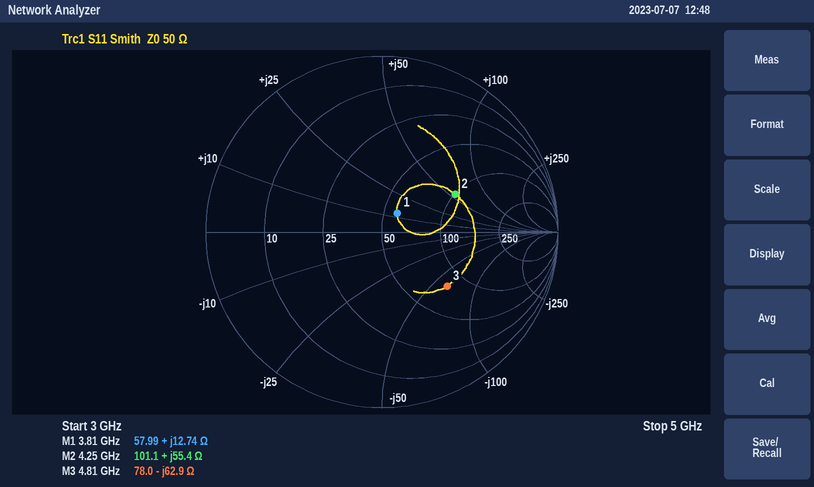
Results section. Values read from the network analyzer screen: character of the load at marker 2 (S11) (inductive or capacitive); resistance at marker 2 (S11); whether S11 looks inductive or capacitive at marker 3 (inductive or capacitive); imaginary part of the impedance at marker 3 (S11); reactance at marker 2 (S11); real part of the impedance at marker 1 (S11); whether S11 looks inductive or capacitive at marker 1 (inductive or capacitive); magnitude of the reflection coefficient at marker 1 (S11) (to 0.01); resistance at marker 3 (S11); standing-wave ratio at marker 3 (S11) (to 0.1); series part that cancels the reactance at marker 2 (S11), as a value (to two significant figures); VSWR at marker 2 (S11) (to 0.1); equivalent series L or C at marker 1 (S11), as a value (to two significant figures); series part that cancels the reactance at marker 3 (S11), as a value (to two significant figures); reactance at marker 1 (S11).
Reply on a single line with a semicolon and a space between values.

inductive; 101.1 Ω; capacitive; -62.9 Ω; +55.4 Ω; 57.99 Ω; inductive; 0.14; 78.0 Ω; 2.9; 680 fF; 2.8; 530 pH; 2.1 nH; +12.74 Ω
